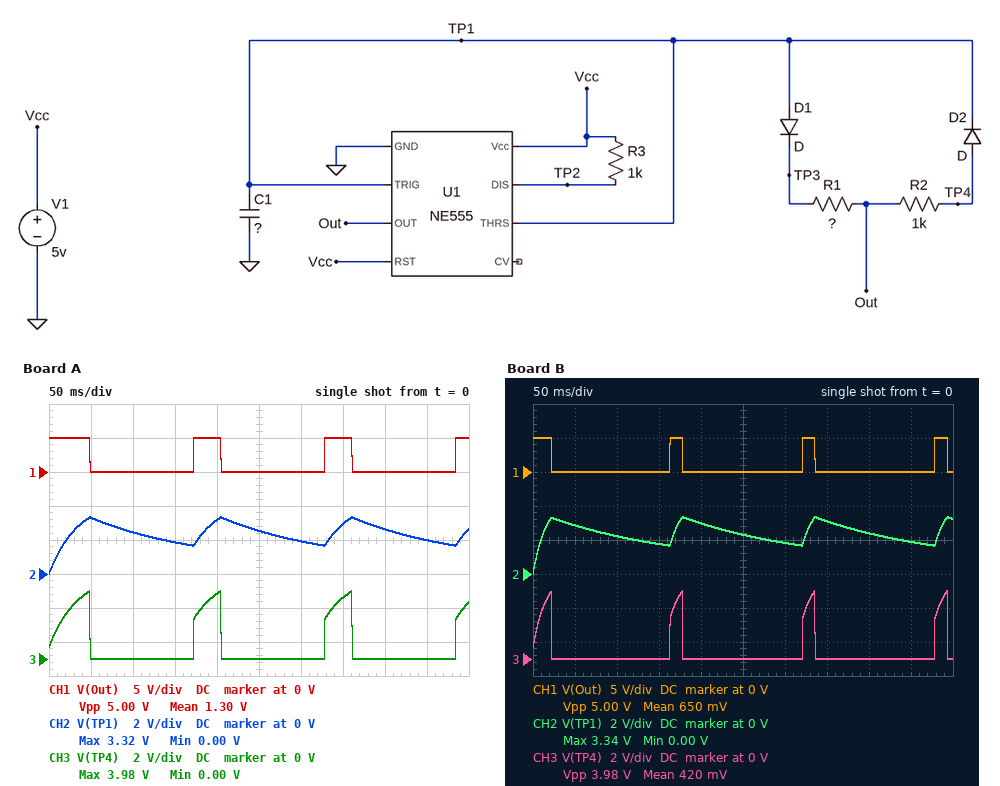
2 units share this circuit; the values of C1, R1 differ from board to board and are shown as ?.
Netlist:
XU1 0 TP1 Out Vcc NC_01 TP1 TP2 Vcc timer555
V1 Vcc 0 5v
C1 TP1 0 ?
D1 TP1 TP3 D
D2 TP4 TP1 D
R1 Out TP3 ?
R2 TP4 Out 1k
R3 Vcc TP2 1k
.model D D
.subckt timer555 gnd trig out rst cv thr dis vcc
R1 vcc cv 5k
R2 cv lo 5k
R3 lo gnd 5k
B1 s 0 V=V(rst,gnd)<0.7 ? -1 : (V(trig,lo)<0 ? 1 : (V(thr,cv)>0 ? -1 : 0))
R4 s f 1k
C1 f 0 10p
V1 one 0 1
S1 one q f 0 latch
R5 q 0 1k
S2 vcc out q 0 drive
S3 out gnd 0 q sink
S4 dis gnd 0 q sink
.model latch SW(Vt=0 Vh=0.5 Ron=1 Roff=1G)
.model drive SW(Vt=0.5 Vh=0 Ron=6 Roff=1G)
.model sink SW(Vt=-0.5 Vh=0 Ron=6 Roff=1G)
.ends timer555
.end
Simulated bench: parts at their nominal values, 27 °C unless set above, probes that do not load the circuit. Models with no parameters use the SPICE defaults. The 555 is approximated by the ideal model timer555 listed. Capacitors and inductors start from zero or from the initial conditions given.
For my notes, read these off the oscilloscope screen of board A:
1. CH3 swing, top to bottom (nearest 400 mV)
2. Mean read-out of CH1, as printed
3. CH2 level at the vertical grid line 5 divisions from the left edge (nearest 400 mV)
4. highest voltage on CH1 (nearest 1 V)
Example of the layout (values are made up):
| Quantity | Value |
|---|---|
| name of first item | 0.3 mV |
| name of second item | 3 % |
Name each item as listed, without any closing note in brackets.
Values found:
| Quantity | Value |
|---|---|
| CH3 swing, top to bottom | 4.0 V |
| Mean read-out of CH1, as printed | 1.30 V |
| CH2 level at the vertical grid line 5 divisions from the left edge | 2.4 V |
| highest voltage on CH1 | 5 V |
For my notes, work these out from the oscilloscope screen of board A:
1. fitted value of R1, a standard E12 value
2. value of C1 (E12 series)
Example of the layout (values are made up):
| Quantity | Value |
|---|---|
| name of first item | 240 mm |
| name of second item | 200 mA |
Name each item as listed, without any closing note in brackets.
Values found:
| Quantity | Value |
|---|---|
| fitted value of R1, a standard E12 value | 3.9 kΩ |
| value of C1 | 33 µF |
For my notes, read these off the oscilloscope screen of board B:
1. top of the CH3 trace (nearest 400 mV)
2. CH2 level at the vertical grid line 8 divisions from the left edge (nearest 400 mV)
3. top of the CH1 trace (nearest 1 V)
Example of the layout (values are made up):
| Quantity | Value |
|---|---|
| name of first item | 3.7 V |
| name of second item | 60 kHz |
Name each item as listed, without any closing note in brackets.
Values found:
| Quantity | Value |
|---|---|
| top of the CH3 trace | 4.0 V |
| CH2 level at the vertical grid line 8 divisions from the left edge | 2.4 V |
| top of the CH1 trace | 5 V |
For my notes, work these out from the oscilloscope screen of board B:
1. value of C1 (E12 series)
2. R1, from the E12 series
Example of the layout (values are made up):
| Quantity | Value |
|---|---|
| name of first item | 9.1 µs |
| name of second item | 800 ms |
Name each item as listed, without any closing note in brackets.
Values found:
| Quantity | Value |
|---|---|
| value of C1 | 15 µF |
| R1, from the E12 series | 10 kΩ |
